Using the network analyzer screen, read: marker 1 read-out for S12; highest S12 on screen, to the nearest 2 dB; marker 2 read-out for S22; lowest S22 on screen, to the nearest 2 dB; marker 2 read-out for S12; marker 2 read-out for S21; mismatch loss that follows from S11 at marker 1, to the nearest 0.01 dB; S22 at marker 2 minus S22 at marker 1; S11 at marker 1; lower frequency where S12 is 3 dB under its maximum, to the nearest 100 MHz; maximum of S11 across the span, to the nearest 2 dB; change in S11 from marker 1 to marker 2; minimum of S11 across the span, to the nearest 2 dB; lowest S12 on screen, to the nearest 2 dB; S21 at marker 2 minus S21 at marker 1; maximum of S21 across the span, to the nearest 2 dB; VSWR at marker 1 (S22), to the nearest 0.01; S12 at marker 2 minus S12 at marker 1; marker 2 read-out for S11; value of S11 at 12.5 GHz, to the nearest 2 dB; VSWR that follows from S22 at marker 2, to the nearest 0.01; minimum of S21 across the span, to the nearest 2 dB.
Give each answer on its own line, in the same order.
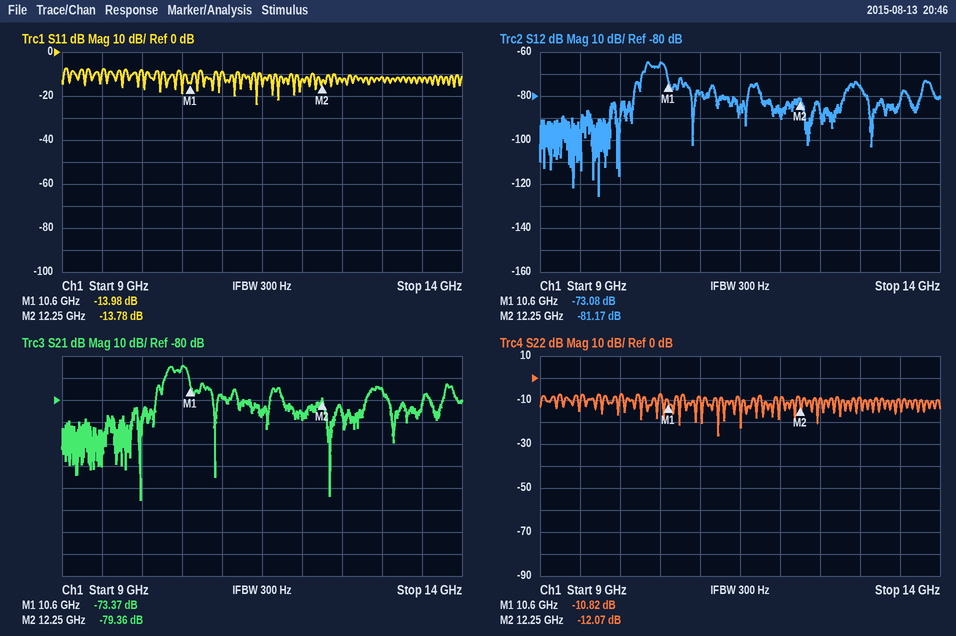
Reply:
-73.08 dB
-64 dB
-12.07 dB
-26 dB
-81.17 dB
-79.36 dB
0.18 dB
-1.25 dB
-13.98 dB
10.3 GHz
-8 dB
0.20 dB
-24 dB
-126 dB
-5.99 dB
-64 dB
1.81
-8.09 dB
-13.78 dB
-14 dB
1.66
-126 dB
